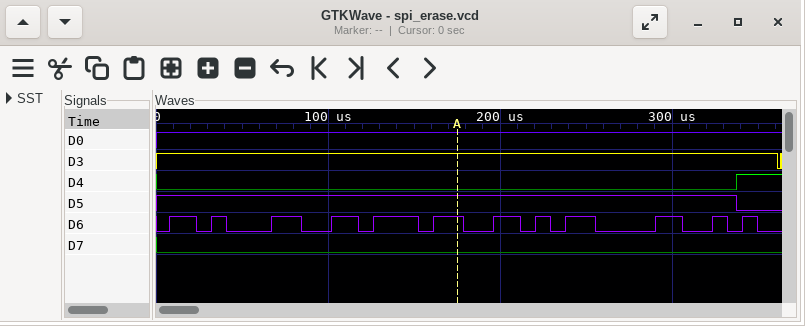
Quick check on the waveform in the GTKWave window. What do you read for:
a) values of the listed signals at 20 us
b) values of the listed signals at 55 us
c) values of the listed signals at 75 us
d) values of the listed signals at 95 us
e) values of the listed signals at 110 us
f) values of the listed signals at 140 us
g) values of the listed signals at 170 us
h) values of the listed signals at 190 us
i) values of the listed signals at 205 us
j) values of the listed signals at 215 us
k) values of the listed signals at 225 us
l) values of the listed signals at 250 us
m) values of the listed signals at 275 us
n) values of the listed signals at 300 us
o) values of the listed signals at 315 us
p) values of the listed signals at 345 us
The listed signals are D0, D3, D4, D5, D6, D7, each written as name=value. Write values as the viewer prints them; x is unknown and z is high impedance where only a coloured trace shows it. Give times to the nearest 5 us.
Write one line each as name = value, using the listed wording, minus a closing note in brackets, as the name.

values of the listed signals at 20 us = D0=1, D3=1, D4=0, D5=1, D6=1, D7=0
values of the listed signals at 55 us = D0=1, D3=1, D4=0, D5=1, D6=0, D7=0
values of the listed signals at 75 us = D0=1, D3=1, D4=0, D5=1, D6=1, D7=0
values of the listed signals at 95 us = D0=1, D3=1, D4=0, D5=1, D6=0, D7=0
values of the listed signals at 110 us = D0=1, D3=1, D4=0, D5=1, D6=1, D7=0
values of the listed signals at 140 us = D0=1, D3=1, D4=0, D5=1, D6=1, D7=0
values of the listed signals at 170 us = D0=1, D3=1, D4=0, D5=1, D6=1, D7=0
values of the listed signals at 190 us = D0=1, D3=1, D4=0, D5=1, D6=0, D7=0
values of the listed signals at 205 us = D0=1, D3=1, D4=0, D5=1, D6=1, D7=0
values of the listed signals at 215 us = D0=1, D3=1, D4=0, D5=1, D6=0, D7=0
values of the listed signals at 225 us = D0=1, D3=1, D4=0, D5=1, D6=1, D7=0
values of the listed signals at 250 us = D0=1, D3=1, D4=0, D5=1, D6=1, D7=0
values of the listed signals at 275 us = D0=1, D3=1, D4=0, D5=1, D6=0, D7=0
values of the listed signals at 300 us = D0=1, D3=1, D4=0, D5=1, D6=1, D7=0
values of the listed signals at 315 us = D0=1, D3=1, D4=0, D5=1, D6=0, D7=0
values of the listed signals at 345 us = D0=1, D3=1, D4=1, D5=0, D6=1, D7=0
